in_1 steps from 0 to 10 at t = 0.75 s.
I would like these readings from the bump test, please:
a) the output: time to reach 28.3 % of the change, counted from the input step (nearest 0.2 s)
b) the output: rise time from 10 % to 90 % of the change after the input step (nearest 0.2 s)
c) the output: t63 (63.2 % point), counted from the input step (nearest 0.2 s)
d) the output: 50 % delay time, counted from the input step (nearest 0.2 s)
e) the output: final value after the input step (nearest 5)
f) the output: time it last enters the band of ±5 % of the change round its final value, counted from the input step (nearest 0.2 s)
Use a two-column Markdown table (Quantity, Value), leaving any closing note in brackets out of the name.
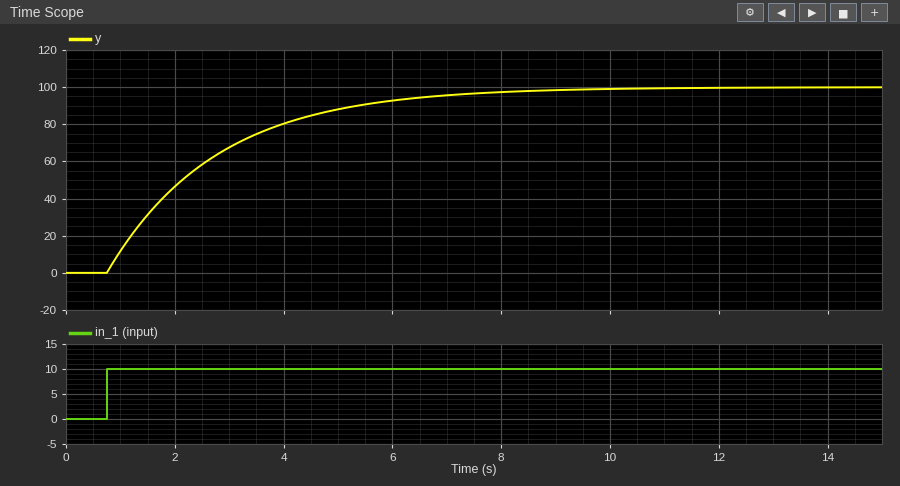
| Quantity | Value |
|---|---|
| the output: time to reach 28.3 % of the change, counted from the input step | 0.6 s |
| the output: rise time from 10 % to 90 % of the change after the input step | 4.4 s |
| the output: t63 (63.2 % point), counted from the input step | 2.0 s |
| the output: 50 % delay time, counted from the input step | 1.4 s |
| the output: final value after the input step | 100 |
| the output: time it last enters the band of ±5 % of the change round its final value, counted from the input step | 6.0 s |
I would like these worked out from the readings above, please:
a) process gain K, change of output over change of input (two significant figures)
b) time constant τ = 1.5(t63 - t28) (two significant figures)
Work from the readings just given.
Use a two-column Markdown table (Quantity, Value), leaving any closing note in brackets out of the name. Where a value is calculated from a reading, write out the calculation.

| Quantity | Value |
|---|---|
| process gain K, change of output over change of input | (100 - 0) / 10 = 10 |
| time constant τ = 1.5(t63 - t28) | 1.5 × (2 - 0.6) = 2.1 s |
